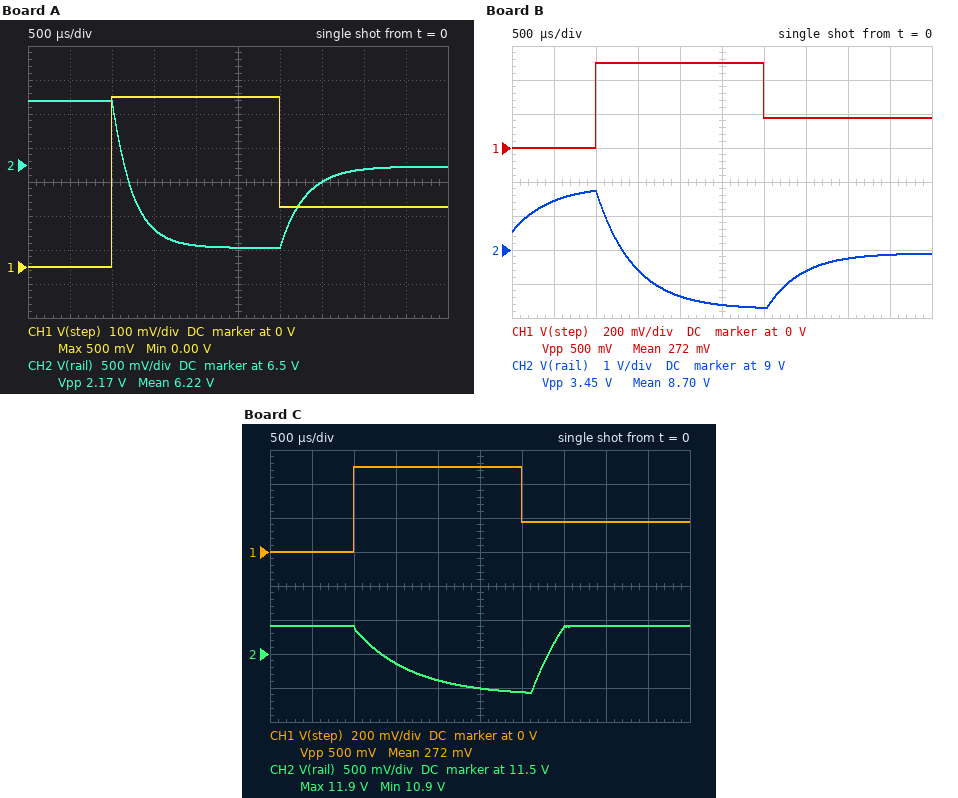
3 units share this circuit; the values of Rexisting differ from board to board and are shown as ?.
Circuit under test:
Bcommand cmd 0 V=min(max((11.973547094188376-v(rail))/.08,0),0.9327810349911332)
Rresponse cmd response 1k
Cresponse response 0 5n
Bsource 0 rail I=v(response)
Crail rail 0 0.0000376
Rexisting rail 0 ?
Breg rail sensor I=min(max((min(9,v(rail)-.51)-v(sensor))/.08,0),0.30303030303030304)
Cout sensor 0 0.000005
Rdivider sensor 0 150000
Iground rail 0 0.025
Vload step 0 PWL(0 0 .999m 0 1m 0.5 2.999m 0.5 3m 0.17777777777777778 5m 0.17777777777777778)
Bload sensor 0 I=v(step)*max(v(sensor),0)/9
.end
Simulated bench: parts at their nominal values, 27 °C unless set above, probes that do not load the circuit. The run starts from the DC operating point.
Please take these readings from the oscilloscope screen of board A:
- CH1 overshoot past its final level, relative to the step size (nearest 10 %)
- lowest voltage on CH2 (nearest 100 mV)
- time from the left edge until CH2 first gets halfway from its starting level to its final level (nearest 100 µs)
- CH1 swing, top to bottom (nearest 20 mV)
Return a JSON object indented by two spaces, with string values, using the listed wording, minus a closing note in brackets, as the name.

{
  "CH1 overshoot past its final level, relative to the step size": "180 %",
  "lowest voltage on CH2": "5.3 V",
  "time from the left edge until CH2 first gets halfway from its starting level to its final level": "1.1 ms",
  "CH1 swing, top to bottom": "500 mV"
}
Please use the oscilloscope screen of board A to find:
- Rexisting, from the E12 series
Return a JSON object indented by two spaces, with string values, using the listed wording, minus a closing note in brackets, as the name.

{
  "Rexisting, from the E12 series": "8.2 Ω"
}
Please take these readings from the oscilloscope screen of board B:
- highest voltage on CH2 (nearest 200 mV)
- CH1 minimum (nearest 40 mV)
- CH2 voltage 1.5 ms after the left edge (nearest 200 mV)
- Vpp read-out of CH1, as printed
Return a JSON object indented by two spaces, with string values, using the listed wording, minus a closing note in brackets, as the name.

{
  "highest voltage on CH2": "10.8 V",
  "CH1 minimum": "0 V",
  "CH2 voltage 1.5 ms after the left edge": "8.4 V",
  "Vpp read-out of CH1, as printed": "500 mV"
}
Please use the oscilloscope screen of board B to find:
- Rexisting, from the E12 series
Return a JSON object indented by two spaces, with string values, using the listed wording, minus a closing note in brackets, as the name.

{
  "Rexisting, from the E12 series": "12 Ω"
}
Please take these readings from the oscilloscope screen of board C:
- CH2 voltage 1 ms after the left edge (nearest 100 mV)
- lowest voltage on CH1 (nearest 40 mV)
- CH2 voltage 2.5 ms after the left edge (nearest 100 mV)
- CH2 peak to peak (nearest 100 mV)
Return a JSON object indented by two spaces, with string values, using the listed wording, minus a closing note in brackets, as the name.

{
  "CH2 voltage 1 ms after the left edge": "11.9 V",
  "lowest voltage on CH1": "0 V",
  "CH2 voltage 2.5 ms after the left edge": "11.0 V",
  "CH2 peak to peak": "1.0 V"
}
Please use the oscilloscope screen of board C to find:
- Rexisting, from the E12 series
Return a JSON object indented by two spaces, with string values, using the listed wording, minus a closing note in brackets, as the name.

{
  "Rexisting, from the E12 series": "18 Ω"
}
